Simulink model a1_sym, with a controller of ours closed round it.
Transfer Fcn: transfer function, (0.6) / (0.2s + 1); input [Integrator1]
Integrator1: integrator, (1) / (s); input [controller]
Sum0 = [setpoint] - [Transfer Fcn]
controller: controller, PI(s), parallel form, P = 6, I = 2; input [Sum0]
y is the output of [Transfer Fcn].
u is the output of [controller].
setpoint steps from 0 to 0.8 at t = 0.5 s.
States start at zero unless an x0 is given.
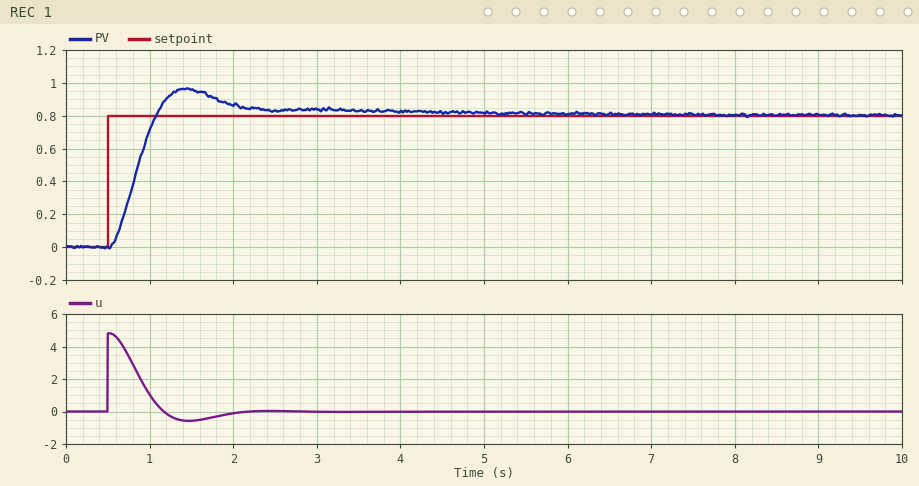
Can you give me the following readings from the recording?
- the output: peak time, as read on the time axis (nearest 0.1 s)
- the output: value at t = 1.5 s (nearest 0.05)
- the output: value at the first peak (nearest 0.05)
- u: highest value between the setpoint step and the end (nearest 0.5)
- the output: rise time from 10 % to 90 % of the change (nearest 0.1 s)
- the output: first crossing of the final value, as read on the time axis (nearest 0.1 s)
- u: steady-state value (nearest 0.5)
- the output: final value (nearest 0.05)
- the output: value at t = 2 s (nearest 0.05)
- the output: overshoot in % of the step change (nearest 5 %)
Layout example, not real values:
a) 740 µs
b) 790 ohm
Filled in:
a) 1.4 s
b) 0.95
c) 0.95
d) 5.0
e) 0.4 s
f) 1.1 s
g) 0.0
h) 0.80
i) 0.85
j) 20 %
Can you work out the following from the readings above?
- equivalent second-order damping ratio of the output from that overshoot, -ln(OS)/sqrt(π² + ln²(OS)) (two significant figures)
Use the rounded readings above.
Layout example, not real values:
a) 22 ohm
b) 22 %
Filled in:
a) 0.46
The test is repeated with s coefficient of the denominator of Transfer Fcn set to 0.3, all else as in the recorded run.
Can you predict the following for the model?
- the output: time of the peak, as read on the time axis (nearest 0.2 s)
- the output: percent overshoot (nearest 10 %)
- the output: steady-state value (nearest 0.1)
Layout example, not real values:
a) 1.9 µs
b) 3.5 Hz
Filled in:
a) 1.6 s
b) 30 %
c) 0.8
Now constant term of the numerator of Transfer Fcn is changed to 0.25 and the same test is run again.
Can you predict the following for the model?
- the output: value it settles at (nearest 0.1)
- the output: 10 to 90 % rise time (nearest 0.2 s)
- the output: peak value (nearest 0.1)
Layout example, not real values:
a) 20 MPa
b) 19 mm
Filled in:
a) 0.8
b) 0.8 s
c) 0.9
